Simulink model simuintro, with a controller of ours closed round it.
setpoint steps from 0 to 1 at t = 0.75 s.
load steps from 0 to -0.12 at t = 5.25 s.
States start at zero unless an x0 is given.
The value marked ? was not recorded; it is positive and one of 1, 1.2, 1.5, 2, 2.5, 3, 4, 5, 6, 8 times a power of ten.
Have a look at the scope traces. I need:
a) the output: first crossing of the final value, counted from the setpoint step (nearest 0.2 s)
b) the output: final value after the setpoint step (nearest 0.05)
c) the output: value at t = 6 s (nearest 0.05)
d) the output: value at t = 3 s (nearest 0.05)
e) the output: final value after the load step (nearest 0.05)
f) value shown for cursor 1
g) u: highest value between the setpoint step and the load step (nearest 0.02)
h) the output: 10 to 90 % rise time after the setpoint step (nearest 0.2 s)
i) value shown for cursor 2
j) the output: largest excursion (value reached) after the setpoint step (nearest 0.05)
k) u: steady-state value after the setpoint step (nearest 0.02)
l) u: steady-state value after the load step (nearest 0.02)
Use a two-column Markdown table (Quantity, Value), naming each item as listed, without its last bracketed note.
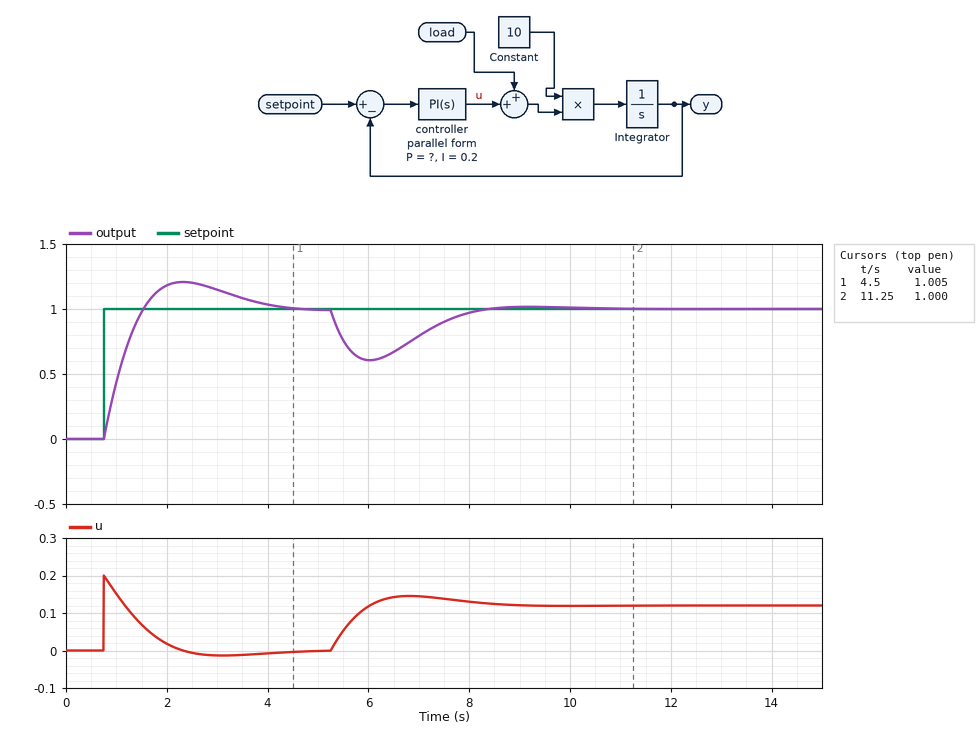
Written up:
| Quantity | Value |
|---|---|
| the output: first crossing of the final value, counted from the setpoint step | 0.8 s |
| the output: final value after the setpoint step | 1.00 |
| the output: value at t = 6 s | 0.60 |
| the output: value at t = 3 s | 1.15 |
| the output: final value after the load step | 1.00 |
| value shown for cursor 1 | 1.005 |
| u: highest value between the setpoint step and the load step | 0.20 |
| the output: 10 to 90 % rise time after the setpoint step | 0.6 s |
| value shown for cursor 2 | 1.000 |
| the output: largest excursion (value reached) after the setpoint step | 1.20 |
| u: steady-state value after the setpoint step | 0.00 |
| u: steady-state value after the load step | 0.12 |
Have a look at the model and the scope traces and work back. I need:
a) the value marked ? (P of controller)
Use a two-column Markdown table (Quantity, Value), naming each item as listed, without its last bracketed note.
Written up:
| Quantity | Value |
|---|---|
| the value marked ? | 0.2 |
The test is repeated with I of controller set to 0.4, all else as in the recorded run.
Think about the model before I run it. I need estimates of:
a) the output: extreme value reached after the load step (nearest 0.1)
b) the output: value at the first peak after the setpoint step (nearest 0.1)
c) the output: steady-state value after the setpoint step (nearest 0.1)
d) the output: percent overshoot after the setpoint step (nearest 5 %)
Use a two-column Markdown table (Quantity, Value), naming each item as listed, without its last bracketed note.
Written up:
| Quantity | Value |
|---|---|
| the output: extreme value reached after the load step | 0.7 |
| the output: value at the first peak after the setpoint step | 1.3 |
| the output: steady-state value after the setpoint step | 1.0 |
| the output: percent overshoot after the setpoint step | 30 % |
